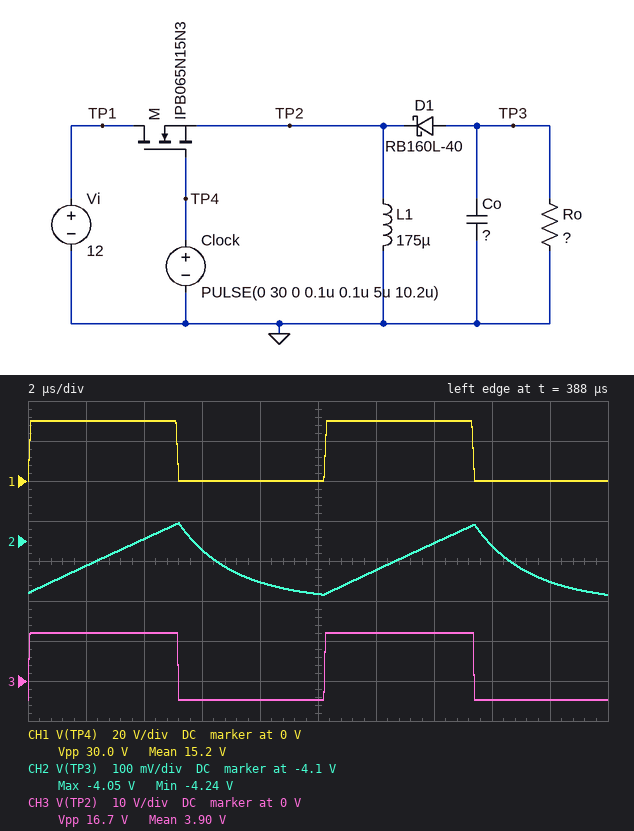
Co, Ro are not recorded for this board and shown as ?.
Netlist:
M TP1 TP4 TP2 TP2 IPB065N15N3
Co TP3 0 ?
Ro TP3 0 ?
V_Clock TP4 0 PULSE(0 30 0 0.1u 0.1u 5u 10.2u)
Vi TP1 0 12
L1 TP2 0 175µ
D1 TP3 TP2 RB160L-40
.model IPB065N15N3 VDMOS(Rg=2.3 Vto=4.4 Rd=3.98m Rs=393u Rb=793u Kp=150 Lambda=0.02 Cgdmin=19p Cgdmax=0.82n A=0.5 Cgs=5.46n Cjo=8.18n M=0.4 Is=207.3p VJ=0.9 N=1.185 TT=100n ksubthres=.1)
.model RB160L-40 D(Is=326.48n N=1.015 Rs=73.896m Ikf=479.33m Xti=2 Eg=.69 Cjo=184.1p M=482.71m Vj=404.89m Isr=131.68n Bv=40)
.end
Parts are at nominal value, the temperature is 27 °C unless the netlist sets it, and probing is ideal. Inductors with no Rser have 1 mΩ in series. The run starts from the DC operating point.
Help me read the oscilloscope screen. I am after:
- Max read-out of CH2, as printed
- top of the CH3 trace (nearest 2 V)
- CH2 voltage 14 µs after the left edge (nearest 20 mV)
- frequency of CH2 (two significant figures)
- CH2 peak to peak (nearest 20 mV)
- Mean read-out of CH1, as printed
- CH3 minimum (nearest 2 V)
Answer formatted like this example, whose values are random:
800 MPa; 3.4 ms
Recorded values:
-4.05 V; 12 V; -4.10 V; 97 kHz; 180 mV; 15.2 V; -4 V
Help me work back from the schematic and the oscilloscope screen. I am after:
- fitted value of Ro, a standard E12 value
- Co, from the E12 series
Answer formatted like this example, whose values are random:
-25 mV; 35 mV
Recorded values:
8.2 Ω; 15 µF
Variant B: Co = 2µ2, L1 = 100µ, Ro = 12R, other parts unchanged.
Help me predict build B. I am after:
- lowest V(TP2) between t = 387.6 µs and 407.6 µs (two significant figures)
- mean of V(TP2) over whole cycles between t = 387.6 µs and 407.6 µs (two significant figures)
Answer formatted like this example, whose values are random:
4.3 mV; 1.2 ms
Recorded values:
-4.8 V; 3.6 V
